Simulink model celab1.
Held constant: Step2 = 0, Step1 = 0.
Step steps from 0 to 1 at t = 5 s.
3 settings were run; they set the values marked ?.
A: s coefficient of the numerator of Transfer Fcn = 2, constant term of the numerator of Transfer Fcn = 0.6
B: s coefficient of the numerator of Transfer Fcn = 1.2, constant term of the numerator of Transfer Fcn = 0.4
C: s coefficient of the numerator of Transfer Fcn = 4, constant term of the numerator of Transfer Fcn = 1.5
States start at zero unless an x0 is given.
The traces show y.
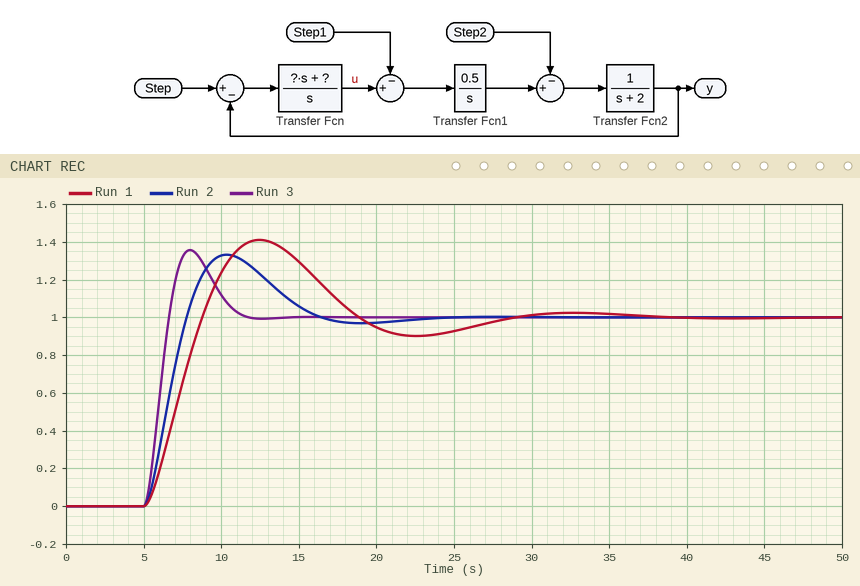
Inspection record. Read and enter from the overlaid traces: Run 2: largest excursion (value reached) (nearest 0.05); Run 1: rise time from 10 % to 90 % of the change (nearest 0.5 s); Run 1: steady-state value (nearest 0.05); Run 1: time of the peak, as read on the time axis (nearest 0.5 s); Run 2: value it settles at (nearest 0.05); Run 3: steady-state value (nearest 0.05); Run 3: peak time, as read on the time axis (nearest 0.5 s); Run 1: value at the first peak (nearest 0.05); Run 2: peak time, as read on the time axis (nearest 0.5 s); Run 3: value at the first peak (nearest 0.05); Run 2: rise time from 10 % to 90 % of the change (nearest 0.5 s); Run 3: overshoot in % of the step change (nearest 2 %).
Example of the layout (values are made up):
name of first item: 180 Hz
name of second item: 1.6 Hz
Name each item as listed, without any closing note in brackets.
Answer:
Run 2: largest excursion (value reached): 1.35
Run 1: rise time from 10 % to 90 % of the change: 2.5 s
Run 1: steady-state value: 1.00
Run 1: time of the peak, as read on the time axis: 12.5 s
Run 2: value it settles at: 1.00
Run 3: steady-state value: 1.00
Run 3: peak time, as read on the time axis: 8.0 s
Run 1: value at the first peak: 1.40
Run 2: peak time, as read on the time axis: 10.5 s
Run 3: value at the first peak: 1.35
Run 2: rise time from 10 % to 90 % of the change: 2.0 s
Run 3: overshoot in % of the step change: 36 %
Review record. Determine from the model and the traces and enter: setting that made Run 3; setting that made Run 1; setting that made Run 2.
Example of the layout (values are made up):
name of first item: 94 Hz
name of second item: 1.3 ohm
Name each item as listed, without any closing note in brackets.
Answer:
setting that made Run 3: C
setting that made Run 1: B
setting that made Run 2: A
